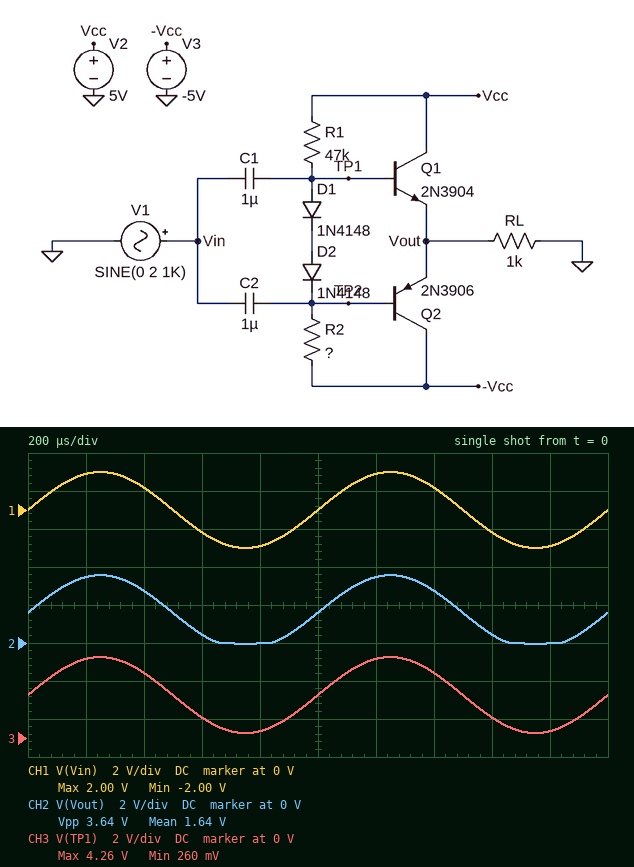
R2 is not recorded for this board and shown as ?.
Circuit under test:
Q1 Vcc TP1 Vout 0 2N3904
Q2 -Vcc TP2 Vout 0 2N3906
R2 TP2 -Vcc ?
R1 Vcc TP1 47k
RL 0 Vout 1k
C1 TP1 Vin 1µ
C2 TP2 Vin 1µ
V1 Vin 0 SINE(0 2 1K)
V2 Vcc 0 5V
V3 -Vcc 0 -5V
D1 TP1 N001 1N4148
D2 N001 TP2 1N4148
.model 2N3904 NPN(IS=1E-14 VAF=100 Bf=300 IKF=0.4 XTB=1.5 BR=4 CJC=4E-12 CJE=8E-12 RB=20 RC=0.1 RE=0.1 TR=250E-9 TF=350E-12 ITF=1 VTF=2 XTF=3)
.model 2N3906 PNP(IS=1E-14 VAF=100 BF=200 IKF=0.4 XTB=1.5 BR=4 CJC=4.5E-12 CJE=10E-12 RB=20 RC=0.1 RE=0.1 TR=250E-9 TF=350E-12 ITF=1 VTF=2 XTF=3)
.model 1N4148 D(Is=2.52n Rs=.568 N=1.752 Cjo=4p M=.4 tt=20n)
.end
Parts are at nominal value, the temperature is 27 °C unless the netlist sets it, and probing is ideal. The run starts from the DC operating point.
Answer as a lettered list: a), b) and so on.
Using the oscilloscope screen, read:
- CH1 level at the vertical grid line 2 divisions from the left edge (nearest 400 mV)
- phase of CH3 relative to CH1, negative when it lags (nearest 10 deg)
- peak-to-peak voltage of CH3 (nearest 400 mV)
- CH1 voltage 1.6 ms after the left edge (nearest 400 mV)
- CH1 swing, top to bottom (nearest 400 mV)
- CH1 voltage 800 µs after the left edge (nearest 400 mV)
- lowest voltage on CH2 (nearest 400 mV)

a) 1.2 V
b) 0 deg
c) 4.0 V
d) -1.2 V
e) 4.0 V
f) -2.0 V
g) 0 V
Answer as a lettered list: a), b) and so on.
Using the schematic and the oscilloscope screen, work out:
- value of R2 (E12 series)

a) 120 kΩ
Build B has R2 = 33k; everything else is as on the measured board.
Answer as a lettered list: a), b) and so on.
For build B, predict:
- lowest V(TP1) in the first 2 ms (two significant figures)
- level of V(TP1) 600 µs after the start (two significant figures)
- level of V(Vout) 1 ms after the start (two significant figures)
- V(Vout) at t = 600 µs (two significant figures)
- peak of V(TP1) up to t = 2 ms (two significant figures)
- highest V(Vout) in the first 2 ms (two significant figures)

a) -2.3 V
b) -1.4 V
c) -580 mV
d) -1.7 V
e) 1.7 V
f) 1.1 V
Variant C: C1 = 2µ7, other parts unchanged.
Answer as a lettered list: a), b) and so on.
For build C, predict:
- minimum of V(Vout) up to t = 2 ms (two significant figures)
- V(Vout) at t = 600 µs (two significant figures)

a) -60 mV
b) 450 mV
